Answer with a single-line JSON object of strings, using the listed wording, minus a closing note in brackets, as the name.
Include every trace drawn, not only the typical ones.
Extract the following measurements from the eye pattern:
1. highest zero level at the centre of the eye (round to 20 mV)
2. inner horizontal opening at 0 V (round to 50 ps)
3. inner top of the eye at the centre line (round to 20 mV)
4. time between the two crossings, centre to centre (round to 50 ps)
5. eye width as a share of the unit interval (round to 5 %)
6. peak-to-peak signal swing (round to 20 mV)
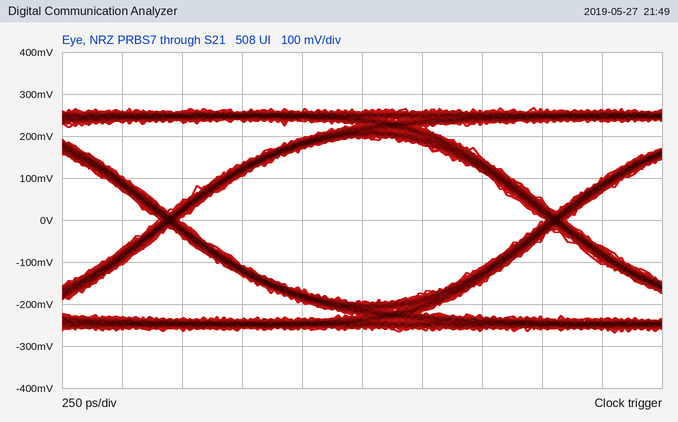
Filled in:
{"highest zero level at the centre of the eye": "-200 mV", "inner horizontal opening at 0 V": "1.55 ns", "inner top of the eye at the centre line": "200 mV", "time between the two crossings, centre to centre": "1.60 ns", "eye width as a share of the unit interval": "95 %", "peak-to-peak signal swing": "540 mV"}
